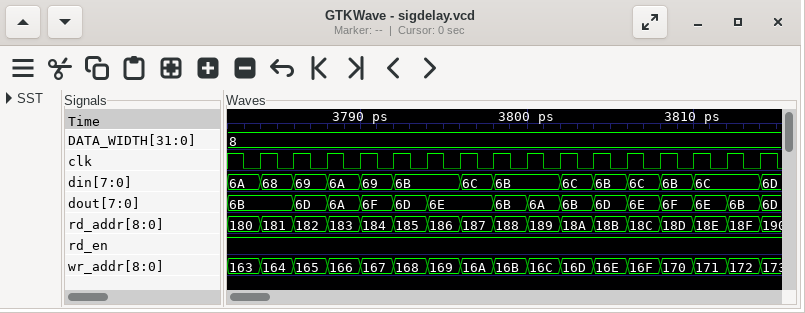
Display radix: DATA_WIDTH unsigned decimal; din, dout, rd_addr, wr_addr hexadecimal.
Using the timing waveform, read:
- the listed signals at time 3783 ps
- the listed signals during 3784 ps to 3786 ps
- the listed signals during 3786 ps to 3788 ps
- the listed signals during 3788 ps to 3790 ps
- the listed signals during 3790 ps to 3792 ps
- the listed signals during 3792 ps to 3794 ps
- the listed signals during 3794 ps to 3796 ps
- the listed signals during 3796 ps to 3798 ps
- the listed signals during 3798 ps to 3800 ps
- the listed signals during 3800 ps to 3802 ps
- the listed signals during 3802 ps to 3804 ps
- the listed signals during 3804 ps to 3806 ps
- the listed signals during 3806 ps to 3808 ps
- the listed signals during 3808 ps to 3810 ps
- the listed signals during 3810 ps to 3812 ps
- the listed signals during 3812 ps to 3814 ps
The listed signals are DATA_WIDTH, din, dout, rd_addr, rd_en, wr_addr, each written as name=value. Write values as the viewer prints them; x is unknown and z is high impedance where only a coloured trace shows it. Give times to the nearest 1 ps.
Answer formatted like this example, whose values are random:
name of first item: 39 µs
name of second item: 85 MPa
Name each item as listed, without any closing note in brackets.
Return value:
the listed signals at time 3783 ps: DATA_WIDTH=8, din=6A, dout=6B, rd_addr=180, rd_en=1, wr_addr=163
the listed signals during 3784 ps to 3786 ps: DATA_WIDTH=8, din=68, dout=6B, rd_addr=181, rd_en=1, wr_addr=164
the listed signals during 3786 ps to 3788 ps: DATA_WIDTH=8, din=69, dout=6D, rd_addr=182, rd_en=1, wr_addr=165
the listed signals during 3788 ps to 3790 ps: DATA_WIDTH=8, din=6A, dout=6A, rd_addr=183, rd_en=1, wr_addr=166
the listed signals during 3790 ps to 3792 ps: DATA_WIDTH=8, din=69, dout=6F, rd_addr=184, rd_en=1, wr_addr=167
the listed signals during 3792 ps to 3794 ps: DATA_WIDTH=8, din=6B, dout=6D, rd_addr=185, rd_en=1, wr_addr=168
the listed signals during 3794 ps to 3796 ps: DATA_WIDTH=8, din=6B, dout=6E, rd_addr=186, rd_en=1, wr_addr=169
the listed signals during 3796 ps to 3798 ps: DATA_WIDTH=8, din=6C, dout=6E, rd_addr=187, rd_en=1, wr_addr=16A
the listed signals during 3798 ps to 3800 ps: DATA_WIDTH=8, din=6B, dout=6B, rd_addr=188, rd_en=1, wr_addr=16B
the listed signals during 3800 ps to 3802 ps: DATA_WIDTH=8, din=6B, dout=6A, rd_addr=189, rd_en=1, wr_addr=16C
the listed signals during 3802 ps to 3804 ps: DATA_WIDTH=8, din=6C, dout=6B, rd_addr=18A, rd_en=1, wr_addr=16D
the listed signals during 3804 ps to 3806 ps: DATA_WIDTH=8, din=6B, dout=6D, rd_addr=18B, rd_en=1, wr_addr=16E
the listed signals during 3806 ps to 3808 ps: DATA_WIDTH=8, din=6C, dout=6E, rd_addr=18C, rd_en=1, wr_addr=16F
the listed signals during 3808 ps to 3810 ps: DATA_WIDTH=8, din=6B, dout=6F, rd_addr=18D, rd_en=1, wr_addr=170
the listed signals during 3810 ps to 3812 ps: DATA_WIDTH=8, din=6C, dout=6E, rd_addr=18E, rd_en=1, wr_addr=171
the listed signals during 3812 ps to 3814 ps: DATA_WIDTH=8, din=6C, dout=6B, rd_addr=18F, rd_en=1, wr_addr=172
